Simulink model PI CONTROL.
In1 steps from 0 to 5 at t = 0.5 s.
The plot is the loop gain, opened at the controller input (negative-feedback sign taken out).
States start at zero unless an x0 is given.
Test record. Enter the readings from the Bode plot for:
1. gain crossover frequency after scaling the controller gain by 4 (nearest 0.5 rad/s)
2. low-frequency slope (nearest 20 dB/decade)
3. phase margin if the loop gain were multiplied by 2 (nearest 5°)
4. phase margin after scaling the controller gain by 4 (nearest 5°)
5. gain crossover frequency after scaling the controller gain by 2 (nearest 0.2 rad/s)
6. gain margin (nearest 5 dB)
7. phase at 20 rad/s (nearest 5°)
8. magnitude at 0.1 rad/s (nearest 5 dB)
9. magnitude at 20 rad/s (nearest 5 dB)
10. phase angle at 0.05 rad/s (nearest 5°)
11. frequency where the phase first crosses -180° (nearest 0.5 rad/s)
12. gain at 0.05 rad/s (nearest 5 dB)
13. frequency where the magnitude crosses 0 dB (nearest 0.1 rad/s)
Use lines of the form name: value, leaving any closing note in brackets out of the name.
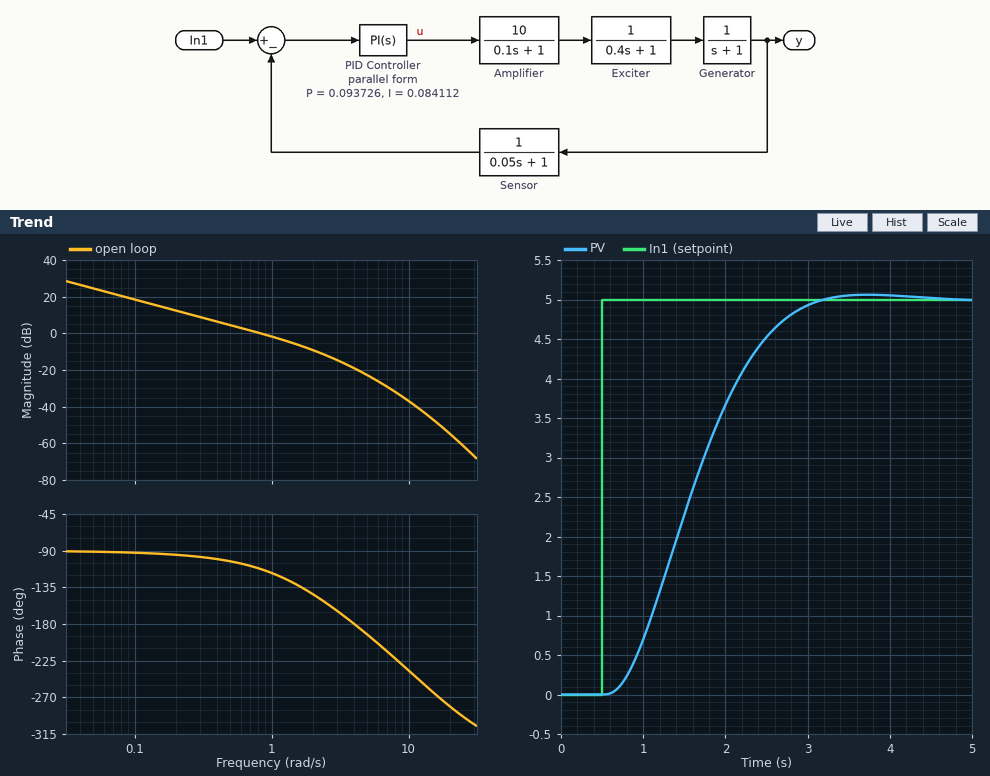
gain crossover frequency after scaling the controller gain by 4: 2.5 rad/s
low-frequency slope: -20 dB/decade
phase margin if the loop gain were multiplied by 2: 50°
phase margin after scaling the controller gain by 4: 25°
gain crossover frequency after scaling the controller gain by 2: 1.6 rad/s
gain margin: 20 dB
phase at 20 rad/s: -280°
magnitude at 0.1 rad/s: 20 dB
magnitude at 20 rad/s: -55 dB
phase angle at 0.05 rad/s: -90°
frequency where the phase first crosses -180°: 4.0 rad/s
gain at 0.05 rad/s: 25 dB
frequency where the magnitude crosses 0 dB: 0.8 rad/s
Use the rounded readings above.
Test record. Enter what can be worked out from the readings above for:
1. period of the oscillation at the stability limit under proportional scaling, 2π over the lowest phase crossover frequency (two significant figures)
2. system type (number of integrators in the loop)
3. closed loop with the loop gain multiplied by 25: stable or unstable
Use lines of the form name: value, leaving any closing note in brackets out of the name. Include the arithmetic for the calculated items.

period of the oscillation at the stability limit under proportional scaling, 2π over the lowest phase crossover frequency: 2π / 4 = 1.6 s
system type: 1
closed loop with the loop gain multiplied by 25: stable or unstable: unstable
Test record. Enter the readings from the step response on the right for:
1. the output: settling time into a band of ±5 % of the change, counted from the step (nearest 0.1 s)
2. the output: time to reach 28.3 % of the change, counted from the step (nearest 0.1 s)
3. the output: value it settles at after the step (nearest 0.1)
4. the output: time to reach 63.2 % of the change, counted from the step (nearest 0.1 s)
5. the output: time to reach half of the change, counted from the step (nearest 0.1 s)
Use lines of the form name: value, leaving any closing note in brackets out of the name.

the output: settling time into a band of ±5 % of the change, counted from the step: 2.2 s
the output: time to reach 28.3 % of the change, counted from the step: 0.7 s
the output: value it settles at after the step: 5.0
the output: time to reach 63.2 % of the change, counted from the step: 1.3 s
the output: time to reach half of the change, counted from the step: 1.1 s
